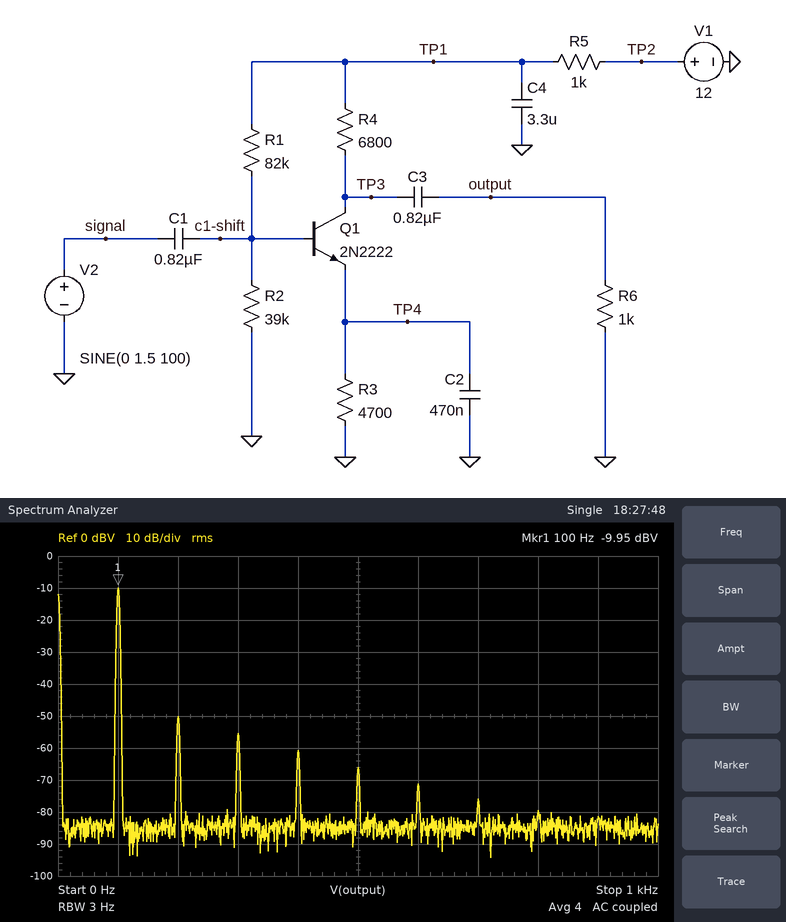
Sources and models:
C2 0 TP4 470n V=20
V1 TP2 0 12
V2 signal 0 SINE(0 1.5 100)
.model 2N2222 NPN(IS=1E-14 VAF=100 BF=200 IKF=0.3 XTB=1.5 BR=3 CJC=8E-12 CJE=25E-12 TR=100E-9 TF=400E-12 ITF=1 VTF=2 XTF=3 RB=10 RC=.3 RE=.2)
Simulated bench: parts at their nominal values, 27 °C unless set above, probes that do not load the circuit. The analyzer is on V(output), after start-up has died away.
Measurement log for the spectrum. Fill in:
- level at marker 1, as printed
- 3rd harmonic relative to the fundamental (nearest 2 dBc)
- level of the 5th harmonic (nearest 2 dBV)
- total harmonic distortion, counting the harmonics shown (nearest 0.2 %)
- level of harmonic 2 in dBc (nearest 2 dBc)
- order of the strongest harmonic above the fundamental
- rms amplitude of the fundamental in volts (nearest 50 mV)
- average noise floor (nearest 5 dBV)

-9.95 dBV
-46 dBc
-66 dBV
1.2 %
-40 dBc
2
300 mV
-85 dBV
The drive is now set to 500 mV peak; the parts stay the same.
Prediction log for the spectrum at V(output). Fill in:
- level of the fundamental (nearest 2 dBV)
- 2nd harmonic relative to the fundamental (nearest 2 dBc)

-20 dBV
-54 dBc
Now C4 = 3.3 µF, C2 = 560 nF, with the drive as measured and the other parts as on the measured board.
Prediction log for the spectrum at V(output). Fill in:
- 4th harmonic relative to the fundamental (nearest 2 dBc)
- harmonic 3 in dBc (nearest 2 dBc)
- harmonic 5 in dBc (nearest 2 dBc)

-42 dBc
-38 dBc
-46 dBc
